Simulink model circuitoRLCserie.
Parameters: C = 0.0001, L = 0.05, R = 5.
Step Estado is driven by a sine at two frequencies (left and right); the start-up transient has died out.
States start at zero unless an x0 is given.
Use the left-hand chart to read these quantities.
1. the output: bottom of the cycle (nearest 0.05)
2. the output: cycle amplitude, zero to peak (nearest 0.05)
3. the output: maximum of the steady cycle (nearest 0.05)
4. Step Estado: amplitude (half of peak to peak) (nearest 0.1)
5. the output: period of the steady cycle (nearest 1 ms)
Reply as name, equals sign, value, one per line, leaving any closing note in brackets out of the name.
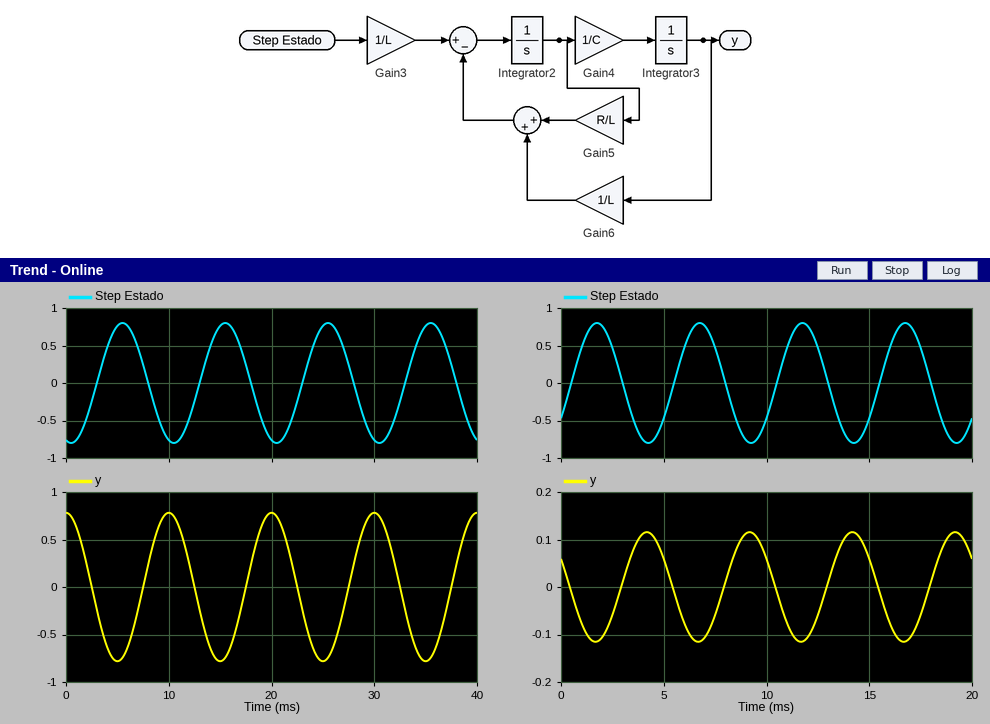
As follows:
the output: bottom of the cycle = -0.80
the output: cycle amplitude, zero to peak = 0.80
the output: maximum of the steady cycle = 0.80
Step Estado: amplitude (half of peak to peak) = 0.8
the output: period of the steady cycle = 10 ms
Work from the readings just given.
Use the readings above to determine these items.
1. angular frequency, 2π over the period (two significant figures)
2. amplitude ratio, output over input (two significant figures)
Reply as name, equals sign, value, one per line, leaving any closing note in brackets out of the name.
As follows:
angular frequency, 2π over the period = 0.63 rad/ms
amplitude ratio, output over input = 1.0
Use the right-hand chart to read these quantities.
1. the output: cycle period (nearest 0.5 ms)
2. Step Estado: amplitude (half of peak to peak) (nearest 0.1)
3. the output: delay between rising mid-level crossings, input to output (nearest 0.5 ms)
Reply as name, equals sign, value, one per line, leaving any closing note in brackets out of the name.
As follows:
the output: cycle period = 5.0 ms
Step Estado: amplitude (half of peak to peak) = 0.8
the output: delay between rising mid-level crossings, input to output = 2.5 ms
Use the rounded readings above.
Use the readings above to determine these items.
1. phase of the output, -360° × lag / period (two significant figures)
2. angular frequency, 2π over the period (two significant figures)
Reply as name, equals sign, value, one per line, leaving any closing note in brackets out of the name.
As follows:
phase of the output, -360° × lag / period = -180°
angular frequency, 2π over the period = 1.3 rad/ms
